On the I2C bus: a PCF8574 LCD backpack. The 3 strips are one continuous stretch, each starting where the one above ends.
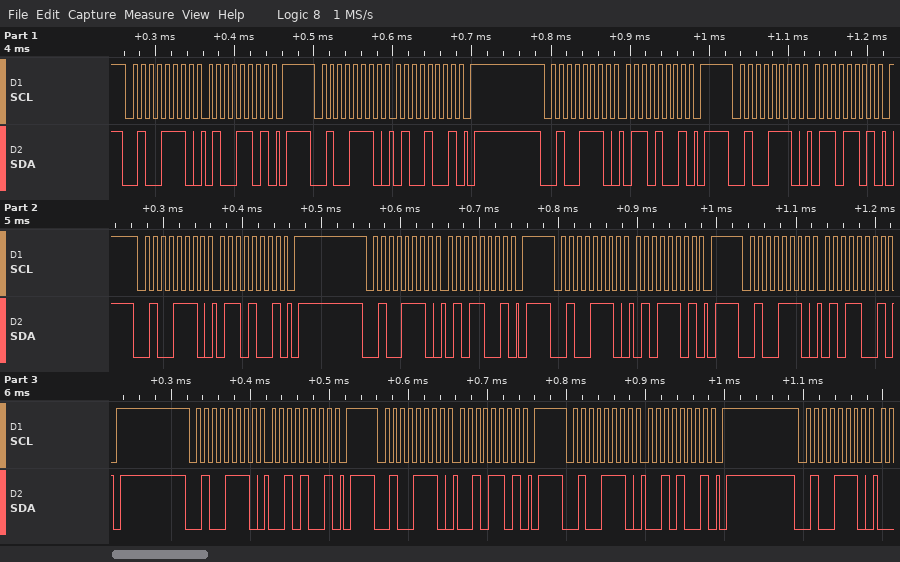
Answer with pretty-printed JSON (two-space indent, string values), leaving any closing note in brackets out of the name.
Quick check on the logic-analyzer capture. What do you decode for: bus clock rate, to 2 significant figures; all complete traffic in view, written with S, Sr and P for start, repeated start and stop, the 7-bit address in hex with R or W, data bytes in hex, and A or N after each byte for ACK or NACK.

{
  "bus clock rate, to 2 significant figures": "100 kHz",
  "all complete traffic in view, written with S, Sr and P for start, repeated start and stop, the 7-bit address in hex with R or W, data bytes in hex, and A or N after each byte for ACK or NACK": "S 27W A 4D A P S 27W A 49 A P S 27W A 69 A P S 27W A 6D A P S 27W A 69 A P S 27W A 59 A P S 27W A 5D A P S 27W A 59 A P S 27W A 29 A P S 27W A 2D A P S 27W A 29 A P S 27W A"
}
